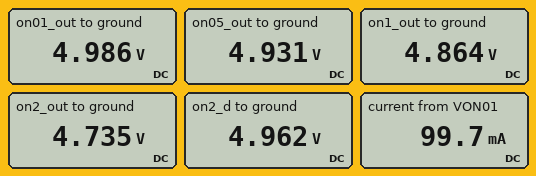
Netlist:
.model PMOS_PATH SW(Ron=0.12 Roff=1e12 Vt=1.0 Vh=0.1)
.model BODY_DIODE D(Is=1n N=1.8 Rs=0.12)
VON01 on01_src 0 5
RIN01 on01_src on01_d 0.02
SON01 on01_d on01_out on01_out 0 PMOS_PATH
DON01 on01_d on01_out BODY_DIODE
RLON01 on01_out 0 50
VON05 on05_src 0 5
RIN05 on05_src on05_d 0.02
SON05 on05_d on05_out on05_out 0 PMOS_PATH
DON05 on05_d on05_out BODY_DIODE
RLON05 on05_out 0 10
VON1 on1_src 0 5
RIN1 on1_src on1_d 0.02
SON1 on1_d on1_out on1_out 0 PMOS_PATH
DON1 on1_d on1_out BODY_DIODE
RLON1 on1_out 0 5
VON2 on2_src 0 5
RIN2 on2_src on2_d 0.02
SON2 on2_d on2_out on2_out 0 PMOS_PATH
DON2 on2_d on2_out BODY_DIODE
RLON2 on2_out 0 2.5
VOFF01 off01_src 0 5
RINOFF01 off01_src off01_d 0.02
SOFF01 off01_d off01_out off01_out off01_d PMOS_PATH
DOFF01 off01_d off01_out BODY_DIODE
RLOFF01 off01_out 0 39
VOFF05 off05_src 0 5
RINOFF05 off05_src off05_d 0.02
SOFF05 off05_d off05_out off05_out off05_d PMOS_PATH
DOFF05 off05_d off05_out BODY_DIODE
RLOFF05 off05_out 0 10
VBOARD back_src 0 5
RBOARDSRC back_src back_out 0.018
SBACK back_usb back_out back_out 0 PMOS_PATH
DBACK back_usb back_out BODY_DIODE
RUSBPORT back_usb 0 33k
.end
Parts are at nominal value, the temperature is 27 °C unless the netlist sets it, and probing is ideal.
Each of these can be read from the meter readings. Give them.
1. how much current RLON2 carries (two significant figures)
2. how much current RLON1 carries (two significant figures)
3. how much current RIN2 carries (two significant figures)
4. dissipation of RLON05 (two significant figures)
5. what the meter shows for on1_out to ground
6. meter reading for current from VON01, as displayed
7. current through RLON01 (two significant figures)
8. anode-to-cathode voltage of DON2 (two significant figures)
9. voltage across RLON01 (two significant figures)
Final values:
1.9 A
970 mA
1.9 A
2.4 W
4.864 V
99.7 mA
100 mA
230 mV
5.0 V
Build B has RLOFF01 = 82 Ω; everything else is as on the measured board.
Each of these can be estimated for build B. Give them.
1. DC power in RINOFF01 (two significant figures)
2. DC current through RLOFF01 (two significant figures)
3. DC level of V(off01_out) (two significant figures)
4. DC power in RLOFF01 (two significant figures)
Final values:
52 µW
51 mA
4.2 V
210 mW
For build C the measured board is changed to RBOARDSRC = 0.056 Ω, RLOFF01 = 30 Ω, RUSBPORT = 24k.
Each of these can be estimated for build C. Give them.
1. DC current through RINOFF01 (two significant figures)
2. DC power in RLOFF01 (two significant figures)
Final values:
140 mA
560 mW
